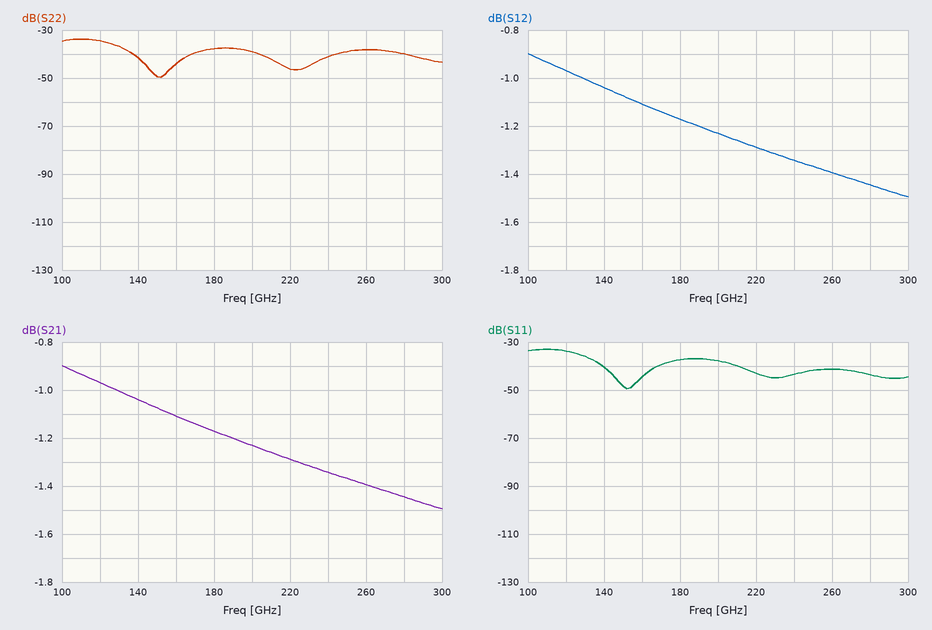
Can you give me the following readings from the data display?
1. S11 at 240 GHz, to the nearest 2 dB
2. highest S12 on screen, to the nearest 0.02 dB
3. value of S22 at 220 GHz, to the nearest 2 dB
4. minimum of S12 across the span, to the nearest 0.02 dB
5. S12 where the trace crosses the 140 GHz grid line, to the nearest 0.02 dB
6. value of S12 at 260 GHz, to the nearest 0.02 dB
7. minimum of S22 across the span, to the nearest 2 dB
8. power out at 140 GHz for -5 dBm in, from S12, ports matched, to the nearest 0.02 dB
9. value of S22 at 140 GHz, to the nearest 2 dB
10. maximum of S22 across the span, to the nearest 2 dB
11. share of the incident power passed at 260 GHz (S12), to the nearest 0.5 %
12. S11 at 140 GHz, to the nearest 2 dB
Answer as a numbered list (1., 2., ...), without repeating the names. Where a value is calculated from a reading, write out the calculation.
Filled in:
1. -44 dB
2. -0.90 dB
3. -46 dB
4. -1.50 dB
5. -1.04 dB
6. -1.40 dB
7. -50 dB
8. -5 dBm + (-1.04 dB) = -6.04 dBm
9. -42 dB
10. -34 dB
11. 10^(-1.4/10) ≈ 72.4 %, so 72.5 % to the nearest 0.5 %
12. -40 dB
